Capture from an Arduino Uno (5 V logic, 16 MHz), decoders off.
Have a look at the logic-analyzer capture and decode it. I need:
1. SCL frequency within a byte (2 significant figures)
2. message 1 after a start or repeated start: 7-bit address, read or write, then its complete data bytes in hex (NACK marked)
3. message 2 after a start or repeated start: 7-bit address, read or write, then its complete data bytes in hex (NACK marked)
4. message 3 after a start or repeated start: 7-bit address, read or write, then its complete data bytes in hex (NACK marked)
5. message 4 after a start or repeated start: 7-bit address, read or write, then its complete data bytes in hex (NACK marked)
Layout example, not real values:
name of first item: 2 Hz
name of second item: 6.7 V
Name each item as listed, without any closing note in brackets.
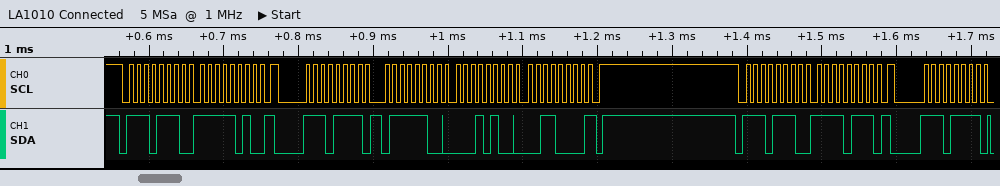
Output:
SCL frequency within a byte: 100 kHz
message 1 after a start or repeated start: 7-bit address, read or write, then its complete data bytes in hex: 0x77 write: FA
message 2 after a start or repeated start: 7-bit address, read or write, then its complete data bytes in hex: 0x77 read: 7C 14 30 NACK
message 3 after a start or repeated start: 7-bit address, read or write, then its complete data bytes in hex: 0x77 write: F7
message 4 after a start or repeated start: 7-bit address, read or write, then its complete data bytes in hex: 0x77 read
